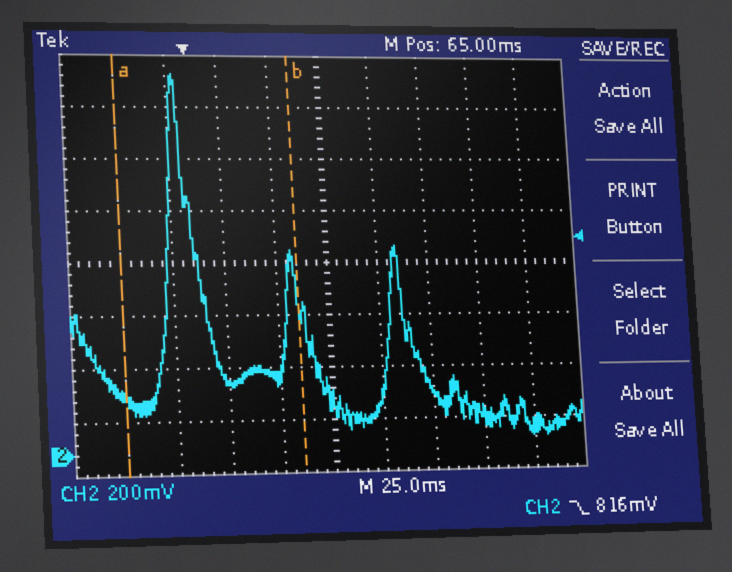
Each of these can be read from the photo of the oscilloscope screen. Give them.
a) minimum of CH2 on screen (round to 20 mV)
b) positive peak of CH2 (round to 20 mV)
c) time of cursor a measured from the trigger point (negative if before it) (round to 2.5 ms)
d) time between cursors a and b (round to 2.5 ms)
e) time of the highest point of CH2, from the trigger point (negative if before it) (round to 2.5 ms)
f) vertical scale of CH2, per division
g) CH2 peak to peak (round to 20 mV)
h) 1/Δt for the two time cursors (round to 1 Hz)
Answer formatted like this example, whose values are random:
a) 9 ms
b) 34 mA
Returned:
a) 40 mV
b) 1.44 V
c) -35.0 ms
d) 85.0 ms
e) -7.5 ms
f) 200 mV
g) 1.40 V
h) 12 Hz
